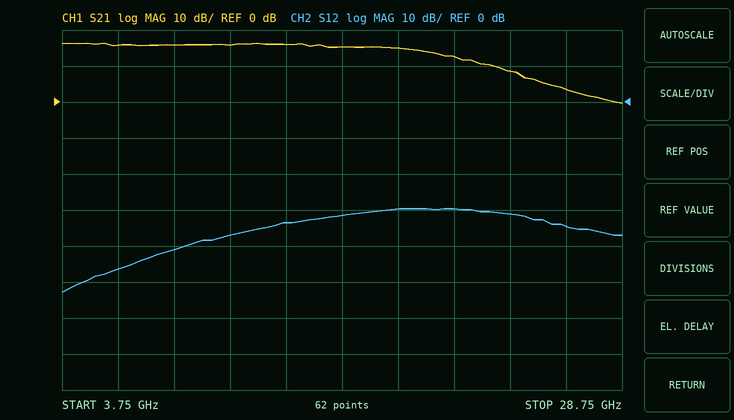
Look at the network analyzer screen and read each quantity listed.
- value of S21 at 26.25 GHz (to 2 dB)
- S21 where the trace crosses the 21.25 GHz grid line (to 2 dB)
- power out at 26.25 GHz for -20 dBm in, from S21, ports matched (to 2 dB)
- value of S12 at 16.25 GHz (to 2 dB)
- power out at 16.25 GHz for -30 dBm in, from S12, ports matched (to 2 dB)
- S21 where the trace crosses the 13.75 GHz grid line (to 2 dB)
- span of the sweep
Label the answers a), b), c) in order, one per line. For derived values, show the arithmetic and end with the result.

a) 4 dB
b) 12 dB
c) -20 dBm + (4 dB) = -16 dBm
d) -32 dB
e) -30 dBm + (-32 dB) = -62 dBm
f) 16 dB
g) 25 GHz
